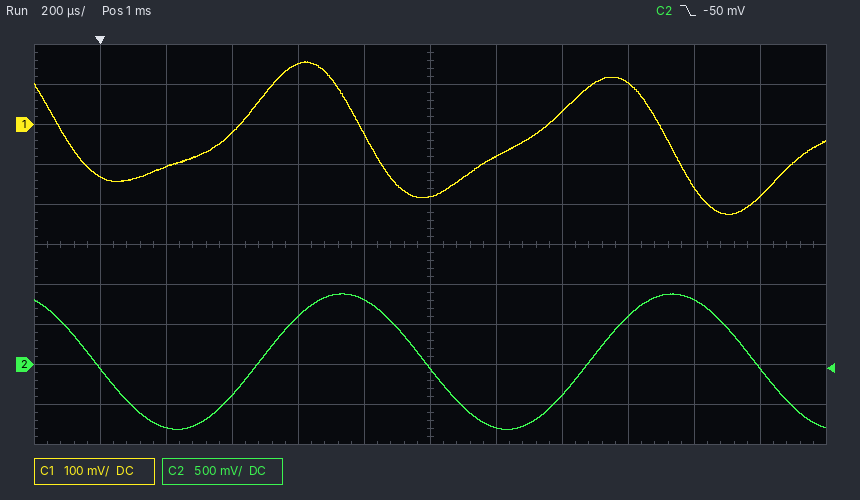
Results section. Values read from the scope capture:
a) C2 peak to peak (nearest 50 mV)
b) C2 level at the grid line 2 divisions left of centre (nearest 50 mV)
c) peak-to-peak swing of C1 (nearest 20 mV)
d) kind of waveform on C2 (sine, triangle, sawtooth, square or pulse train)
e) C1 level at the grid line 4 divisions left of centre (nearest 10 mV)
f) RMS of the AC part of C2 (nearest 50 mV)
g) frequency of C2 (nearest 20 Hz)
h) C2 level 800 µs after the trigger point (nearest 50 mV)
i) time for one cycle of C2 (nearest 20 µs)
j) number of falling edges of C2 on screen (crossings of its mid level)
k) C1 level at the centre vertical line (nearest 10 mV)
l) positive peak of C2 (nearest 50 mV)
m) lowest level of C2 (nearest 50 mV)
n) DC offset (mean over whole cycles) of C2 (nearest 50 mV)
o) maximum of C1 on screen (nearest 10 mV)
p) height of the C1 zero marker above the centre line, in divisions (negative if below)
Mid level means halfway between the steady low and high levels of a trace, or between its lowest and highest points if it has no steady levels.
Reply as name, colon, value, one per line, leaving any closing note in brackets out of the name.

C2 peak to peak: 1.70 V
C2 level at the grid line 2 divisions left of centre: 600 mV
peak-to-peak swing of C1: 380 mV
kind of waveform on C2: sine
C1 level at the grid line 4 divisions left of centre: -110 mV
RMS of the AC part of C2: 600 mV
frequency of C2: 1.00 kHz
C2 level 800 µs after the trigger point: 800 mV
time for one cycle of C2: 1.00 ms
number of falling edges of C2 on screen: 3
C1 level at the centre vertical line: -180 mV
positive peak of C2: 900 mV
lowest level of C2: -800 mV
DC offset (mean over whole cycles) of C2: 50 mV
maximum of C1 on screen: 160 mV
height of the C1 zero marker above the centre line, in divisions: +3.0 div
